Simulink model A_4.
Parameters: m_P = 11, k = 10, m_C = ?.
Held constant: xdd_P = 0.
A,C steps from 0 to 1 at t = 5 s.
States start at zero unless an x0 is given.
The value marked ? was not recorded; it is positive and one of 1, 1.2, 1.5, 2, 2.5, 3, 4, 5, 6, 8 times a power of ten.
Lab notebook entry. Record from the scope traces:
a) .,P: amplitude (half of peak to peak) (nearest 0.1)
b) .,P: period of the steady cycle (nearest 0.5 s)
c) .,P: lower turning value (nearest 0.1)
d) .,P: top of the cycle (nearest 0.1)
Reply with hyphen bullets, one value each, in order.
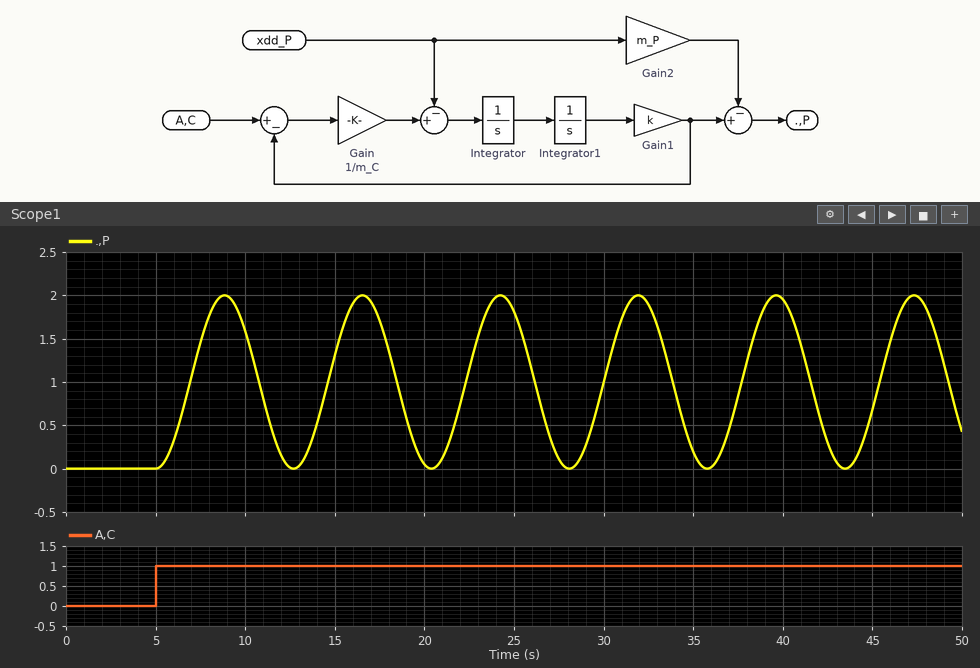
- 1.0
- 7.5 s
- 0.0
- 2.0
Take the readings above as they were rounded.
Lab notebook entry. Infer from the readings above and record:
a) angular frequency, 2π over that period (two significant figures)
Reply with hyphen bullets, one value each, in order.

- 0.84 rad/s
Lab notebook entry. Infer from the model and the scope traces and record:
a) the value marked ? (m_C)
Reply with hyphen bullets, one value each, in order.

- 15
